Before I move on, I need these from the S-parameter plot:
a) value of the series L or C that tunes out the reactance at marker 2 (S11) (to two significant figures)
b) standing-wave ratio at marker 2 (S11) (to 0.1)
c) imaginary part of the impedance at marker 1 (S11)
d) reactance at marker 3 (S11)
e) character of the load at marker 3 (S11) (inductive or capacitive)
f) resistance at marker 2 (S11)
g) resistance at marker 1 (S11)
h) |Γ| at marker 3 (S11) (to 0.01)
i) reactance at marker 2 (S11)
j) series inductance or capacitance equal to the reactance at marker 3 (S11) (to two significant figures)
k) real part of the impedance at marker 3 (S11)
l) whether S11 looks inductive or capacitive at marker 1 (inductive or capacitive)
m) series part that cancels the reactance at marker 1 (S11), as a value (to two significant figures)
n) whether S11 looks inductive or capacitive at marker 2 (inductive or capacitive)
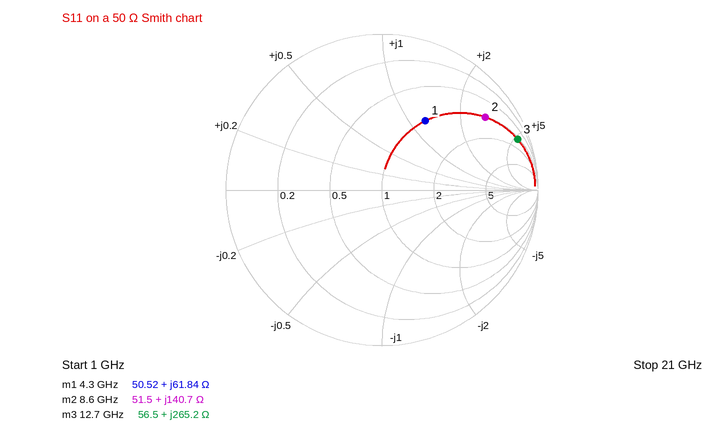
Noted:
130 fF
9.6
+61.84 Ω
+265.2 Ω
inductive
51.5 Ω
50.52 Ω
0.93
+140.7 Ω
3.3 nH
56.5 Ω
inductive
600 fF
inductive
